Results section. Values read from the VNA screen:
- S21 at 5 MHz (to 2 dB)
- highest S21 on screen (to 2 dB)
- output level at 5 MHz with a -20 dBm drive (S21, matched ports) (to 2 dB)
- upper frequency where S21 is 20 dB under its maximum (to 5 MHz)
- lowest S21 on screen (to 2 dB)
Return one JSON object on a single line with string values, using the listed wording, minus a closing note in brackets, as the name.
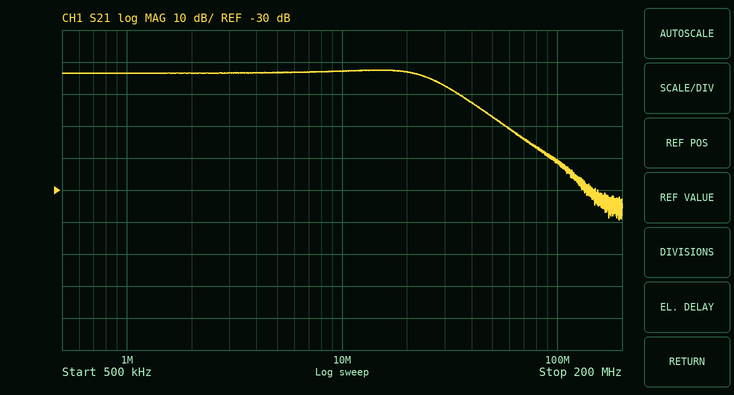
{"S21 at 5 MHz": "6 dB", "highest S21 on screen": "8 dB", "output level at 5 MHz with a -20 dBm drive (S21, matched ports)": "-14 dBm", "upper frequency where S21 is 20 dB under its maximum": "65 MHz", "lowest S21 on screen": "-40 dB"}
